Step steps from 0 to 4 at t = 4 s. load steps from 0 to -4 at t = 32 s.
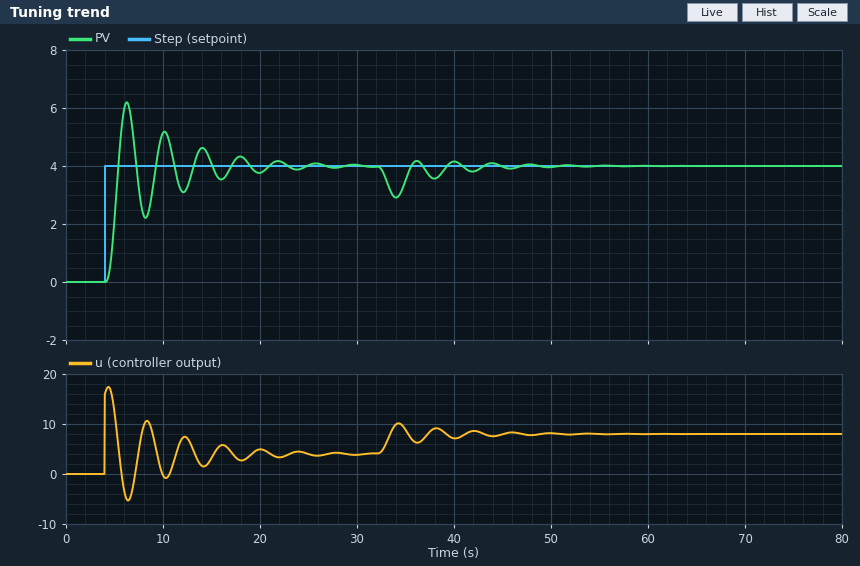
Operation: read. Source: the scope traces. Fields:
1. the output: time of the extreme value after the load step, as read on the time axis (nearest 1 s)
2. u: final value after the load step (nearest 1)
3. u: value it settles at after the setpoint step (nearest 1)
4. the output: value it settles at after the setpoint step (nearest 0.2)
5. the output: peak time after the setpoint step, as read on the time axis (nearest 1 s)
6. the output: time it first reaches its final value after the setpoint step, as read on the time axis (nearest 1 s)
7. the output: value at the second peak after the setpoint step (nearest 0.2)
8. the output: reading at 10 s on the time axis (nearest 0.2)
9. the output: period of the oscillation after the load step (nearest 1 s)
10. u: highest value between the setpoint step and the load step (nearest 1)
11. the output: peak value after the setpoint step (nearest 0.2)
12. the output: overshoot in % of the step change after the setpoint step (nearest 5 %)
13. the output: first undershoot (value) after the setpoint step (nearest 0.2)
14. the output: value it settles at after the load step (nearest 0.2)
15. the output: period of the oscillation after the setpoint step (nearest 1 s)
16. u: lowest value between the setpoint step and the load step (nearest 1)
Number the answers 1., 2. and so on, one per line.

1. 34 s
2. 8
3. 4
4. 4.0
5. 6 s
6. 5 s
7. 5.2
8. 5.2
9. 4 s
10. 17
11. 6.2
12. 55 %
13. 2.2
14. 4.0
15. 4 s
16. -5
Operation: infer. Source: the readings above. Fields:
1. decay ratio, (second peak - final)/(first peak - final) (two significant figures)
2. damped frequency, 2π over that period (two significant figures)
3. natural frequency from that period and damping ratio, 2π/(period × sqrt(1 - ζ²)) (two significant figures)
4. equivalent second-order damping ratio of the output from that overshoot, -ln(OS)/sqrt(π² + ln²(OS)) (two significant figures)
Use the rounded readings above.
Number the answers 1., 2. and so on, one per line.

1. 0.55
2. 1.6 rad/s
3. 1.6 rad/s
4. 0.19
